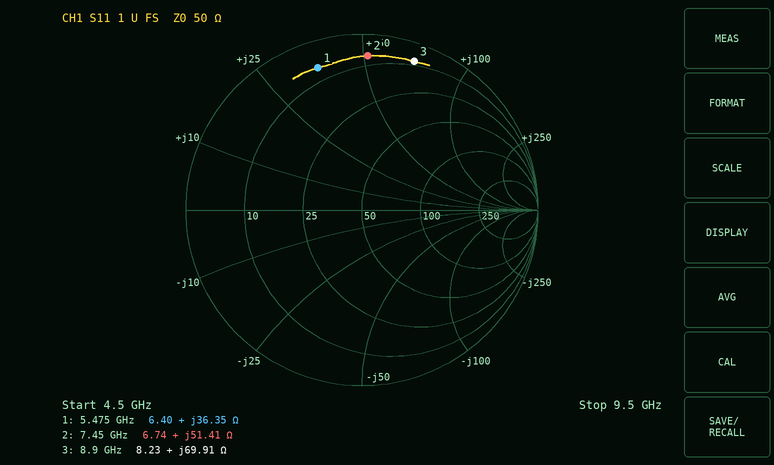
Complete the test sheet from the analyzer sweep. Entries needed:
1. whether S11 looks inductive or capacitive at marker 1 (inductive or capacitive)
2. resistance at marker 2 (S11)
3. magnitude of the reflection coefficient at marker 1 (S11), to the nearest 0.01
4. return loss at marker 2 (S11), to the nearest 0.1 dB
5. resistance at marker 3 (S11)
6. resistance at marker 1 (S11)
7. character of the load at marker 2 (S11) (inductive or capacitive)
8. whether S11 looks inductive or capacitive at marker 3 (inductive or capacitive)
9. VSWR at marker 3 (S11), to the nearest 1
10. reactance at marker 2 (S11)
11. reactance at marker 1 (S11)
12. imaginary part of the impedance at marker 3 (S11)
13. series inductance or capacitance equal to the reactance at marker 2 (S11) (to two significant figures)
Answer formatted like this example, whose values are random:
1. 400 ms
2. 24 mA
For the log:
1. inductive
2. 6.74 Ω
3. 0.85
4. 1.1 dB
5. 8.23 Ω
6. 6.40 Ω
7. inductive
8. inductive
9. 18
10. +51.41 Ω
11. +36.35 Ω
12. +69.91 Ω
13. 1.1 nH
